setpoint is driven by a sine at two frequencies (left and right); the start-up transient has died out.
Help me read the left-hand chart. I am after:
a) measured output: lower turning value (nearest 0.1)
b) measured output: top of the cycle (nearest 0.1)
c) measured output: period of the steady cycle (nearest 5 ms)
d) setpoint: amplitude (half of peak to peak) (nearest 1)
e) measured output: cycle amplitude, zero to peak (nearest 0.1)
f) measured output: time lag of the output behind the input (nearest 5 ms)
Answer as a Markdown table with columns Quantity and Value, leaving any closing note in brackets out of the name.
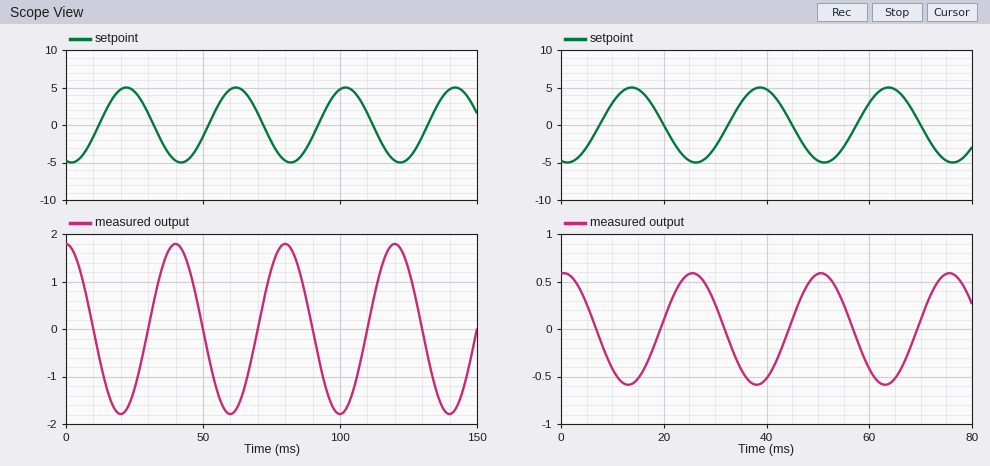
| Quantity | Value |
|---|---|
| measured output: lower turning value | -1.8 |
| measured output: top of the cycle | 1.8 |
| measured output: period of the steady cycle | 40 ms |
| setpoint: amplitude (half of peak to peak) | 5 |
| measured output: cycle amplitude, zero to peak | 1.8 |
| measured output: time lag of the output behind the input | 20 ms |
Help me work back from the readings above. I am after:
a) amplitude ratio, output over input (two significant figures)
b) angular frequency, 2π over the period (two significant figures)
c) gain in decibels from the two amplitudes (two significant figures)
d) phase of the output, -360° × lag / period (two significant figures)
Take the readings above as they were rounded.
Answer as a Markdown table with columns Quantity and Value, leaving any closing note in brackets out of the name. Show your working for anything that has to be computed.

| Quantity | Value |
|---|---|
| amplitude ratio, output over input | 1.8 / 5 = 0.36 |
| angular frequency, 2π over the period | 2π / 40 = 0.16 rad/ms |
| gain in decibels from the two amplitudes | 20 log10(1.8 / 5) = -8.9 dB |
| phase of the output, -360° × lag / period | -360 × 20 / 40 = -180° |
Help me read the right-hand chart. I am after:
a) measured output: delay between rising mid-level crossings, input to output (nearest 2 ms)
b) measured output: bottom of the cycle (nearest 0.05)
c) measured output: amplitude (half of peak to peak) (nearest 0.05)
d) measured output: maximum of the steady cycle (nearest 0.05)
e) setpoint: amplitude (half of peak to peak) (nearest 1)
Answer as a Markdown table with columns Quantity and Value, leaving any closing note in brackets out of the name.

| Quantity | Value |
|---|---|
| measured output: delay between rising mid-level crossings, input to output | 12 ms |
| measured output: bottom of the cycle | -0.60 |
| measured output: amplitude (half of peak to peak) | 0.60 |
| measured output: maximum of the steady cycle | 0.60 |
| setpoint: amplitude (half of peak to peak) | 5 |
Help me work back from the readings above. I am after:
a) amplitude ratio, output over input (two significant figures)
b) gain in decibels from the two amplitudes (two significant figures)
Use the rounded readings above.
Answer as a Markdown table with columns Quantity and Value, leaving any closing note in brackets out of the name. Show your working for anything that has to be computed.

| Quantity | Value |
|---|---|
| amplitude ratio, output over input | 0.6 / 5 = 0.12 |
| gain in decibels from the two amplitudes | 20 log10(0.6 / 5) = -18 dB |
